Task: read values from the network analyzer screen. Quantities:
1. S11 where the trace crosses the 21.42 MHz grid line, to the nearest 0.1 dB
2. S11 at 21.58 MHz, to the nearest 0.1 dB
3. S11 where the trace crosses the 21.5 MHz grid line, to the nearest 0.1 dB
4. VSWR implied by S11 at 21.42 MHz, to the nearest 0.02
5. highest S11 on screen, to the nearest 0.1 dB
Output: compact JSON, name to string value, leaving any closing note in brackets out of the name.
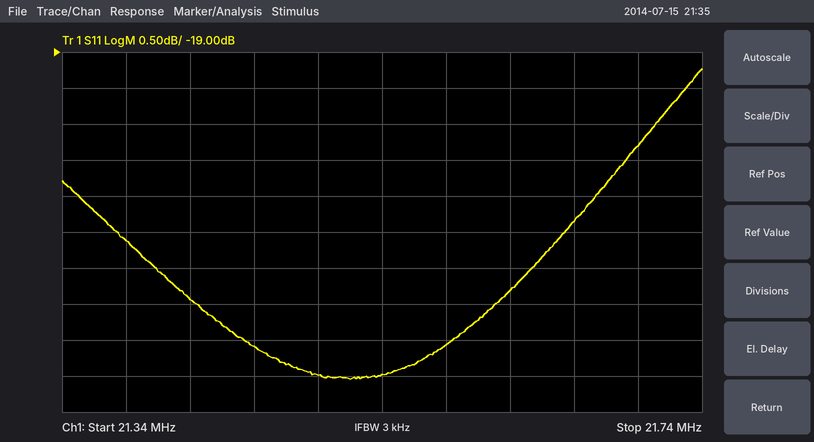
{"S11 where the trace crosses the 21.42 MHz grid line, to the nearest 0.1 dB": "-22.4 dB", "S11 at 21.58 MHz, to the nearest 0.1 dB": "-23.1 dB", "S11 where the trace crosses the 21.5 MHz grid line, to the nearest 0.1 dB": "-23.5 dB", "VSWR implied by S11 at 21.42 MHz, to the nearest 0.02": "1.16", "highest S11 on screen, to the nearest 0.1 dB": "-19.2 dB"}
